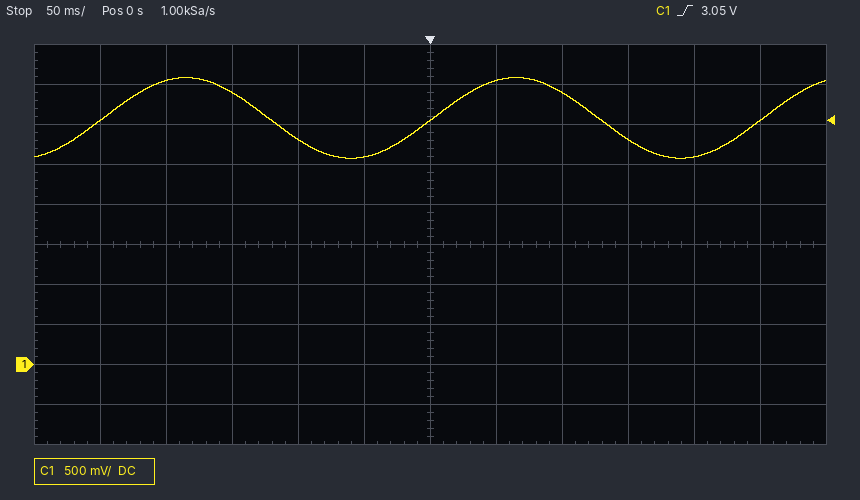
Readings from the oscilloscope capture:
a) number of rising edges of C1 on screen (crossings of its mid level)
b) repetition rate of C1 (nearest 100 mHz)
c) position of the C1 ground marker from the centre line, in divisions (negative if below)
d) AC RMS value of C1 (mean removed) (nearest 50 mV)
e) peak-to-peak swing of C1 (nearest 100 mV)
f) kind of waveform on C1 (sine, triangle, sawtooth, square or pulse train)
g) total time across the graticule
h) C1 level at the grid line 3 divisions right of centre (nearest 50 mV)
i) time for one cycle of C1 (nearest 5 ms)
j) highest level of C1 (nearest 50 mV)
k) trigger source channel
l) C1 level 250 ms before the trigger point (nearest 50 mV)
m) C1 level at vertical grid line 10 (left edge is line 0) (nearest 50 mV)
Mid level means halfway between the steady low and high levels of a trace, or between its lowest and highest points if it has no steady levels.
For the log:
3
4.0 Hz
-3.0 div
350 mV
1.00 V
sine
600 ms
2.80 V
250 ms
3.60 V
C1
3.05 V
2.60 V
